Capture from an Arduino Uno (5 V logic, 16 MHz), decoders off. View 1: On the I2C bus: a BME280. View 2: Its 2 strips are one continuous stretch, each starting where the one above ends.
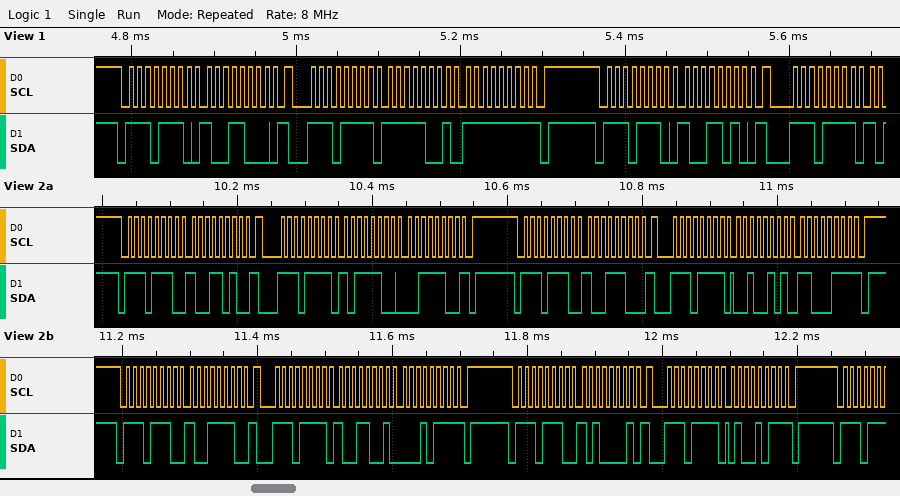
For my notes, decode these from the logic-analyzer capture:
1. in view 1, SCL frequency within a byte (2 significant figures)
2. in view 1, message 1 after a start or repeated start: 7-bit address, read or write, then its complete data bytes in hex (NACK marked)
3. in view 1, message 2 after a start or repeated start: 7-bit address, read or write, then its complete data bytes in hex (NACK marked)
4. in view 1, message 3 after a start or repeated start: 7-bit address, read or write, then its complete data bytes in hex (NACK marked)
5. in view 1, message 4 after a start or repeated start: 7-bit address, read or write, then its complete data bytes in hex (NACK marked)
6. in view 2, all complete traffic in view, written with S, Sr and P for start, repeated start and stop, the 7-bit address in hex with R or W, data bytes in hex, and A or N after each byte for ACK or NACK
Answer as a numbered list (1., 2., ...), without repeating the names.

1. 100 kHz
2. 0x77 write: 98
3. 0x77 read: F9 FF NACK
4. 0x77 write: 9A
5. 0x77 read
6. S 77W A 9A A Sr 77R A BC A 3C N P S 77W A 9C A Sr 77R A 25 A C7 N P S 77W A 9E A Sr 77R A 99 A 17 N P S 77W A A1 A Sr 77R A 4B N P
